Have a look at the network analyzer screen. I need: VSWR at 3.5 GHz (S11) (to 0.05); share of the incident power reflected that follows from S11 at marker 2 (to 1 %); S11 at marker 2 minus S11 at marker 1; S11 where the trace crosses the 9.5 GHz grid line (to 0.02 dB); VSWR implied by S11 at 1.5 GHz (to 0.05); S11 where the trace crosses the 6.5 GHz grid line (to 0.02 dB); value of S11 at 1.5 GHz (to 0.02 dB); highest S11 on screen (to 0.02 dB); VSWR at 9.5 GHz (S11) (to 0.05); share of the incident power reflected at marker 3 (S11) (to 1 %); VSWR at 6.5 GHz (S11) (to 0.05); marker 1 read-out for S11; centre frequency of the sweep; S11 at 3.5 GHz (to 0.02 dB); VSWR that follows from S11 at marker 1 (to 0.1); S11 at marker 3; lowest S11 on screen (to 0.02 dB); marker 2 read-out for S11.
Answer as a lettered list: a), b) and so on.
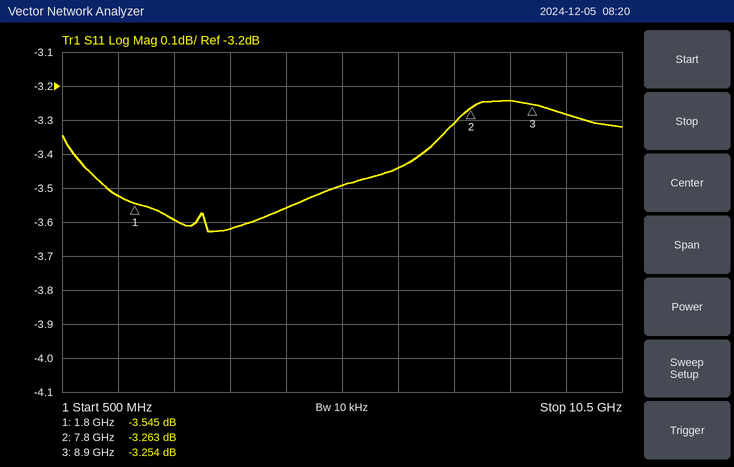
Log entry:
a) 4.85
b) 47 %
c) 0.282 dB
d) -3.28 dB
e) 5.00
f) -3.44 dB
g) -3.52 dB
h) -3.24 dB
i) 5.35
j) 47 %
k) 5.10
l) -3.545 dB
m) 5.5 GHz
n) -3.62 dB
o) 5.0
p) -3.254 dB
q) -3.62 dB
r) -3.263 dB
